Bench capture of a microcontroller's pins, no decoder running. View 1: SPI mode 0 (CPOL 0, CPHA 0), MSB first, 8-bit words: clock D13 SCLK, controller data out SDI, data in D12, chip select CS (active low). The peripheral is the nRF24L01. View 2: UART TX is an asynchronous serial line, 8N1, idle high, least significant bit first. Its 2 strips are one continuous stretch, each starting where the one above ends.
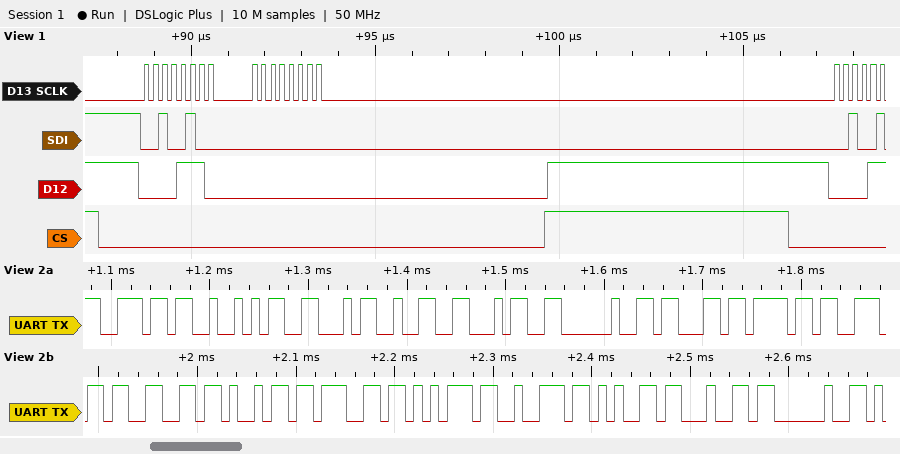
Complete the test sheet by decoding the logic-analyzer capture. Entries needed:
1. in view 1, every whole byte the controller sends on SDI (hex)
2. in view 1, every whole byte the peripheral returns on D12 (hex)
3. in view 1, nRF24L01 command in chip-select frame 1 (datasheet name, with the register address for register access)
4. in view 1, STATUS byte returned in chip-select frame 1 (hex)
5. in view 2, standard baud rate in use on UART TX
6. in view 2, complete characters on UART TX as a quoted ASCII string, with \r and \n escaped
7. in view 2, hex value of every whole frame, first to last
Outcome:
24 00
0E 00
W_REGISTER 0x04
0x0E
115200 baud
"nRF24 configured "
6E 52 46 32 34 20 63 6F 6E 66 69 67 75 72 65 64 20
